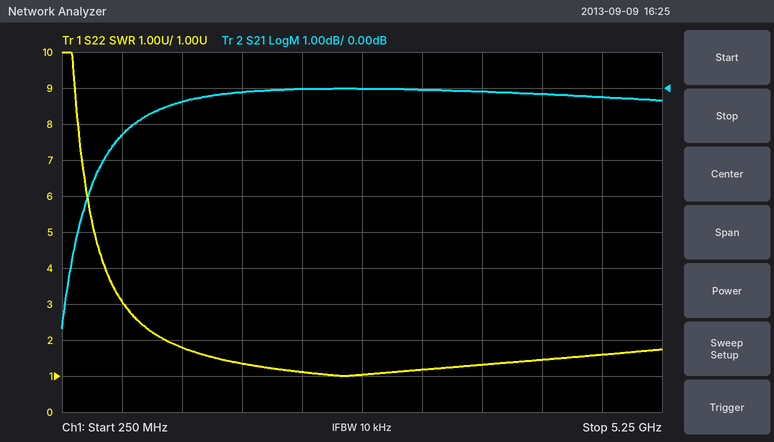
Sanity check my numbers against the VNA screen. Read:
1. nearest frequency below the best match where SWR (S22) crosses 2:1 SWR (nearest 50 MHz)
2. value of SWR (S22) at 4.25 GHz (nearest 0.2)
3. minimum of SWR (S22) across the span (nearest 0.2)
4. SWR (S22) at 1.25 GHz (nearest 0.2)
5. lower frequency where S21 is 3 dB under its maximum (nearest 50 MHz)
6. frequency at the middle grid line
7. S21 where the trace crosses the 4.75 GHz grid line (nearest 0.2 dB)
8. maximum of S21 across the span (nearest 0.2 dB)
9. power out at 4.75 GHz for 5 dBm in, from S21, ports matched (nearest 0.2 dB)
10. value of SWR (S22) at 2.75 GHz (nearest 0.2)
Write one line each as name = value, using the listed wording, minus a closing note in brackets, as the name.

nearest frequency below the best match where SWR (S22) crosses 2:1 SWR = 1.10 GHz
value of SWR (S22) at 4.25 GHz = 1.4
minimum of SWR (S22) across the span = 1.0
SWR (S22) at 1.25 GHz = 1.8
lower frequency where S21 is 3 dB under its maximum = 450 MHz
frequency at the middle grid line = 2.75 GHz
S21 where the trace crosses the 4.75 GHz grid line = -0.2 dB
maximum of S21 across the span = 0.0 dB
power out at 4.75 GHz for 5 dBm in, from S21, ports matched = 4.8 dBm
value of SWR (S22) at 2.75 GHz = 1.0
